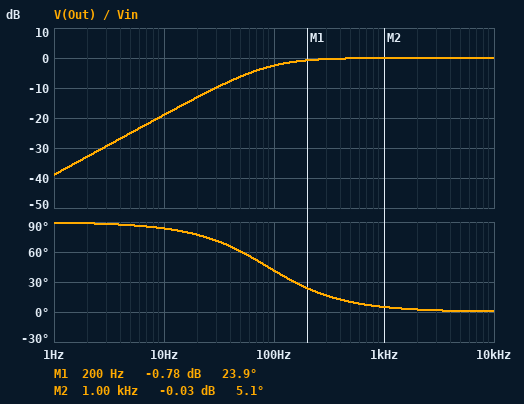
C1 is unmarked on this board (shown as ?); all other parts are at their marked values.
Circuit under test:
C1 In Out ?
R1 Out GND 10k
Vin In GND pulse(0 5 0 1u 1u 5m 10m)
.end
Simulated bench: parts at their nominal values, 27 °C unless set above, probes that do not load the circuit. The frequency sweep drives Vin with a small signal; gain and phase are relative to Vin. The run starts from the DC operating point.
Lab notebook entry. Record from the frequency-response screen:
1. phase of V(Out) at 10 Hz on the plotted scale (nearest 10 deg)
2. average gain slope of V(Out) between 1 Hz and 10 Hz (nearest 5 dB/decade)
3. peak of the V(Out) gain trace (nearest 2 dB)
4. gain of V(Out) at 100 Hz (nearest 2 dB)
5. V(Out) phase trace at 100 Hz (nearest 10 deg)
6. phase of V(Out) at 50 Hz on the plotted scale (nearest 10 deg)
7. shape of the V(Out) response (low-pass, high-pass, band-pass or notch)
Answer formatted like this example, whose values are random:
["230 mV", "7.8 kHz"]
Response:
["80 deg", "20 dB/decade", "0 dB", "-2 dB", "40 deg", "60 deg", "high-pass"]
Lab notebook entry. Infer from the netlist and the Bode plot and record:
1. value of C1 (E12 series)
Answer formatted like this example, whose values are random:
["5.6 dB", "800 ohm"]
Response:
["180 nF"]
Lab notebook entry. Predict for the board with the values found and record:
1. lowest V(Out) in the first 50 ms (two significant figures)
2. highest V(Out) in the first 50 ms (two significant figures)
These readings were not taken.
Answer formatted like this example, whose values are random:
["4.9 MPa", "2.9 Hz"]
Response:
["-4.7 V", "5.0 V"]
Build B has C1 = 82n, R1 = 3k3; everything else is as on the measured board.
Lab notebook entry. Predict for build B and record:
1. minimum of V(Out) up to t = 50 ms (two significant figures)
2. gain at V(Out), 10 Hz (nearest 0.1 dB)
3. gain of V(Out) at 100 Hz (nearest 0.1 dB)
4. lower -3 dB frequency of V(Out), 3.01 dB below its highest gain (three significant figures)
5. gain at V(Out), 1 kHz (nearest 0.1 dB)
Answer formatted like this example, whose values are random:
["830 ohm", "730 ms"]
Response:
["-5.0 V", "-35.4 dB", "-15.5 dB", "588 Hz", "-1.3 dB"]
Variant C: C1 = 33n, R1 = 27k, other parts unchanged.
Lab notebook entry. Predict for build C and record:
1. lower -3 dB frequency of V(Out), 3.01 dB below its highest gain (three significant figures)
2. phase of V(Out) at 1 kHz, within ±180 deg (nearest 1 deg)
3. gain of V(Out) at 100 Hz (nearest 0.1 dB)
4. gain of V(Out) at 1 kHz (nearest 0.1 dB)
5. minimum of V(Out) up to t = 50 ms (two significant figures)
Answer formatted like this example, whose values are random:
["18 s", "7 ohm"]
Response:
["179 Hz", "10 deg", "-6.2 dB", "-0.1 dB", "-5.0 V"]
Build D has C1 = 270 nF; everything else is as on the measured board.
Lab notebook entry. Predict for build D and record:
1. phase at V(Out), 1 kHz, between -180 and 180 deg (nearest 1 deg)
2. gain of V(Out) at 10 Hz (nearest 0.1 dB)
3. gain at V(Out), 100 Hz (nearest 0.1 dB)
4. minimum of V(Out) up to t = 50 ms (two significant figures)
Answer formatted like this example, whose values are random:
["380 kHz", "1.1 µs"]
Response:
["3 deg", "-15.5 dB", "-1.3 dB", "-4.3 V"]
